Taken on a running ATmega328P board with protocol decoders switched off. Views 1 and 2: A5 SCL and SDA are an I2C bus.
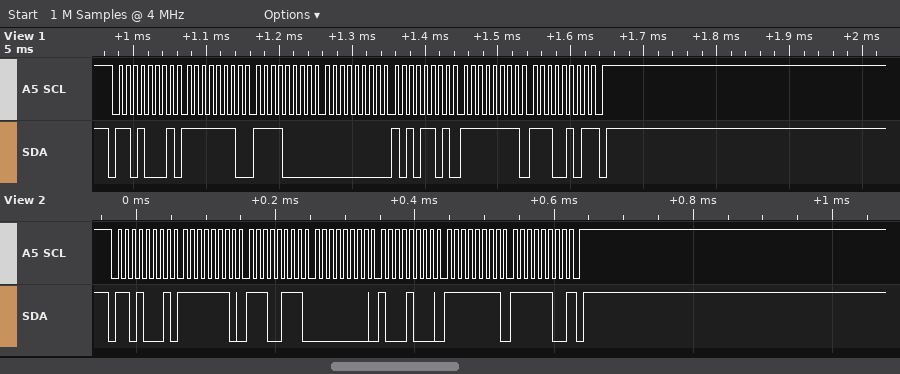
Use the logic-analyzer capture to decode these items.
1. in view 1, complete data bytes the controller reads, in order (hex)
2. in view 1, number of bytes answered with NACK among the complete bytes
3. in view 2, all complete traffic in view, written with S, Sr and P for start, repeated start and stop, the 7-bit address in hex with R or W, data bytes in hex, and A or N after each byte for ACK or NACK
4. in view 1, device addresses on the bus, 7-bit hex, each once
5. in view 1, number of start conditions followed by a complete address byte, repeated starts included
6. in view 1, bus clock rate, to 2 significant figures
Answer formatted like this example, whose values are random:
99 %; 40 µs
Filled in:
FE F0 00 AD FF E5; 1; S 68R A FE A E7 A 00 A 88 A FF A FC N P; 0x68; 1; 100 kHz
